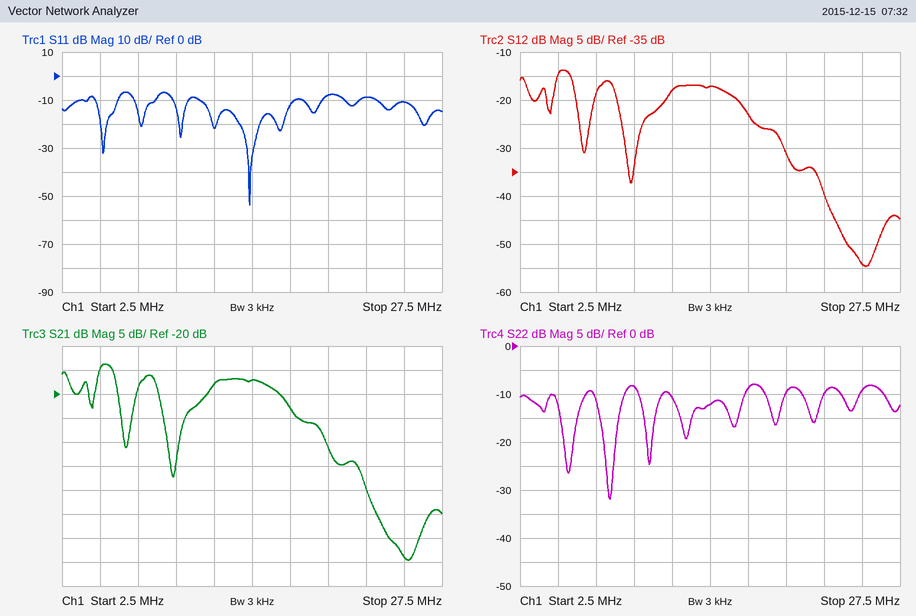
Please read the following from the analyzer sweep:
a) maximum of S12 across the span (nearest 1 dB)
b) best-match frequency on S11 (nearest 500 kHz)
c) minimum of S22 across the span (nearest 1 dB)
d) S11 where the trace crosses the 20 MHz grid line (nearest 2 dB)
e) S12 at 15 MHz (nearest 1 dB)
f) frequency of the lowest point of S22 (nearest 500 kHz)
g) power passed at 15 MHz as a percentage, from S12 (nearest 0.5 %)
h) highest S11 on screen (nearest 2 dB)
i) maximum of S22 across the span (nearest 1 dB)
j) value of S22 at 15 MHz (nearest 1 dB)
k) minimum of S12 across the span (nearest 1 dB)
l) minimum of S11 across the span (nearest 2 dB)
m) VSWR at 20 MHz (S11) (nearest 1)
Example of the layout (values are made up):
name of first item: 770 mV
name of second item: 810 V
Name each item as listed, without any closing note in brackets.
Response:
maximum of S12 across the span: -14 dB
best-match frequency on S11: 15.0 MHz
minimum of S22 across the span: -32 dB
S11 where the trace crosses the 20 MHz grid line: -8 dB
S12 at 15 MHz: -17 dB
frequency of the lowest point of S22: 8.5 MHz
power passed at 15 MHz as a percentage, from S12: 2.0 %
highest S11 on screen: -6 dB
maximum of S22 across the span: -8 dB
value of S22 at 15 MHz: -12 dB
minimum of S12 across the span: -55 dB
minimum of S11 across the span: -54 dB
VSWR at 20 MHz (S11): 2
